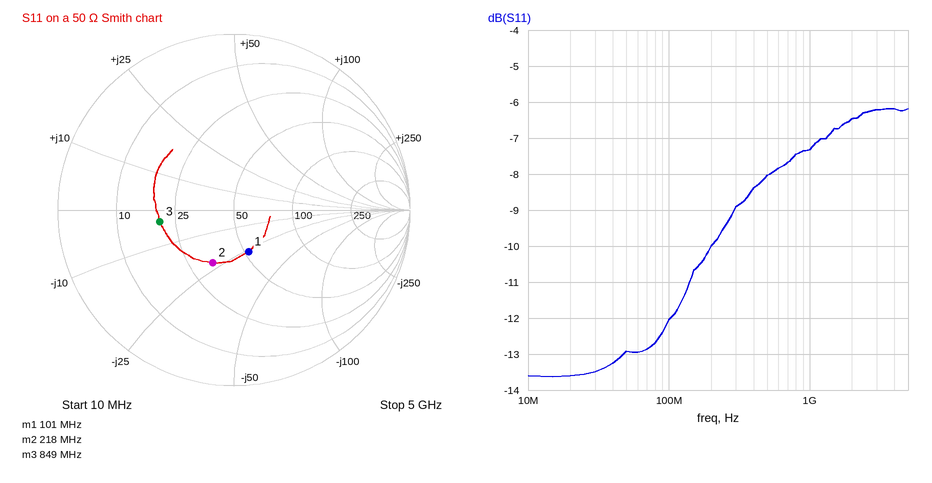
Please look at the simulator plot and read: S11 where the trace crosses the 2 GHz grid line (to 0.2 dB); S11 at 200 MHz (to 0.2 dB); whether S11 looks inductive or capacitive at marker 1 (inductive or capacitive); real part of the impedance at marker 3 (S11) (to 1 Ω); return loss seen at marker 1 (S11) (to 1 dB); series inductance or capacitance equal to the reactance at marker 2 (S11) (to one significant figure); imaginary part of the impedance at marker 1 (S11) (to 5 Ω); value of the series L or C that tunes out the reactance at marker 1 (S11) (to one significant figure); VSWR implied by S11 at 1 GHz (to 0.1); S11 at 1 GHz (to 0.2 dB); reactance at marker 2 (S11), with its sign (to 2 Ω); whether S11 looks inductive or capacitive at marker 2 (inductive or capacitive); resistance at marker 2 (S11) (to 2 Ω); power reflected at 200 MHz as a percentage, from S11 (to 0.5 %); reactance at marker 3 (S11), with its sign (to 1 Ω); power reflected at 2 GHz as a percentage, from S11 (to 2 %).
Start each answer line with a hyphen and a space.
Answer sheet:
- -6.4 dB
- -10.0 dB
- capacitive
- 20 Ω
- 12 dB
- 30 pF
- -25 Ω
- 40 nH
- 2.5
- -7.4 dB
- -22 Ω
- capacitive
- 34 Ω
- 10.0 %
- -3 Ω
- 22 %
